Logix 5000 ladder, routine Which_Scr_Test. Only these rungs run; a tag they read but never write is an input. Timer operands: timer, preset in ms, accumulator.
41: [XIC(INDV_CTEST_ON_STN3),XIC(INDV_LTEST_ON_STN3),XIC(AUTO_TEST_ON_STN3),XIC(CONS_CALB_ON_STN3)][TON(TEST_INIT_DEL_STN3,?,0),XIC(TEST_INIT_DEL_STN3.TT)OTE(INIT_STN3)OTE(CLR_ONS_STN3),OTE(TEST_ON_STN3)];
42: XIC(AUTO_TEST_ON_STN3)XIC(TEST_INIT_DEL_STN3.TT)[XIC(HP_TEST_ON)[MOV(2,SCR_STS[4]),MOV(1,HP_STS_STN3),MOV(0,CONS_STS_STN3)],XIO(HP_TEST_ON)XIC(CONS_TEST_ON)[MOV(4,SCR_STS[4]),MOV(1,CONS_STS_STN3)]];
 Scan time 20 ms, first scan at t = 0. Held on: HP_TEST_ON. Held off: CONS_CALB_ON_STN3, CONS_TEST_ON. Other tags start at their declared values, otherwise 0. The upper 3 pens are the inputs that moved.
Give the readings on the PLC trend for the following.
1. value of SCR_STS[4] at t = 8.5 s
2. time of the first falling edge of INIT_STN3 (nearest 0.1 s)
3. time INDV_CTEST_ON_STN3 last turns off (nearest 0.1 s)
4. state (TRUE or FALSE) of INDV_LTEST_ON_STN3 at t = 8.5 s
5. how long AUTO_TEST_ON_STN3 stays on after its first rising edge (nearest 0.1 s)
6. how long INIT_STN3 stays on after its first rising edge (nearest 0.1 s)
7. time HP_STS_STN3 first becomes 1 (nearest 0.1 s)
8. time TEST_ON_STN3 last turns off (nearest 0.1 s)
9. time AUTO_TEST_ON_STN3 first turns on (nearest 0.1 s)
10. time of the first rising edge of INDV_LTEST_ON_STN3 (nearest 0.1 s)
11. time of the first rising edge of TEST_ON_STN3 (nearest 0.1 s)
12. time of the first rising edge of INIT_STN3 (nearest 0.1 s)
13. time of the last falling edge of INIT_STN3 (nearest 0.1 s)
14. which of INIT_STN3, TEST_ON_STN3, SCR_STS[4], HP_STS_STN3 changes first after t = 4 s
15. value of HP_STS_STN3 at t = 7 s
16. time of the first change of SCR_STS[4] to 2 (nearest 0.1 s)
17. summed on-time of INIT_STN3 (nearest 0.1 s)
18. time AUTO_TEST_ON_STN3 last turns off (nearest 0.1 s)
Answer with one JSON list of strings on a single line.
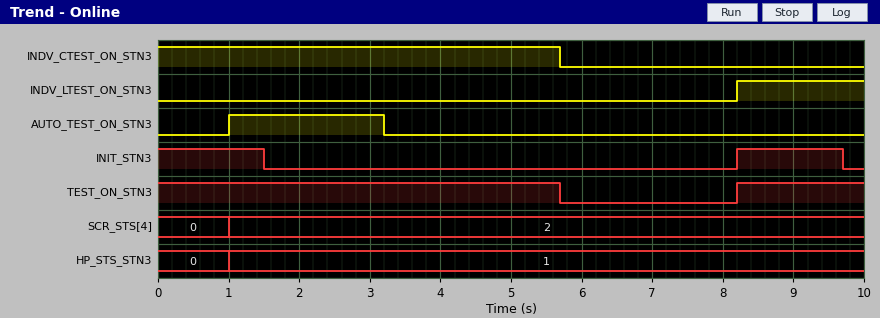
["2", "1.5 s", "5.7 s", "TRUE", "2.2 s", "1.5 s", "1.0 s", "5.7 s", "1.0 s", "8.2 s", "8.2 s", "8.2 s", "9.7 s", "TEST_ON_STN3", "1", "1.0 s", "3.0 s", "3.2 s"]
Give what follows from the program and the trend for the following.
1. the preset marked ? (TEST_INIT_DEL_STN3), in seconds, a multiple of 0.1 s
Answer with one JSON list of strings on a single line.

["1.5 s"]
